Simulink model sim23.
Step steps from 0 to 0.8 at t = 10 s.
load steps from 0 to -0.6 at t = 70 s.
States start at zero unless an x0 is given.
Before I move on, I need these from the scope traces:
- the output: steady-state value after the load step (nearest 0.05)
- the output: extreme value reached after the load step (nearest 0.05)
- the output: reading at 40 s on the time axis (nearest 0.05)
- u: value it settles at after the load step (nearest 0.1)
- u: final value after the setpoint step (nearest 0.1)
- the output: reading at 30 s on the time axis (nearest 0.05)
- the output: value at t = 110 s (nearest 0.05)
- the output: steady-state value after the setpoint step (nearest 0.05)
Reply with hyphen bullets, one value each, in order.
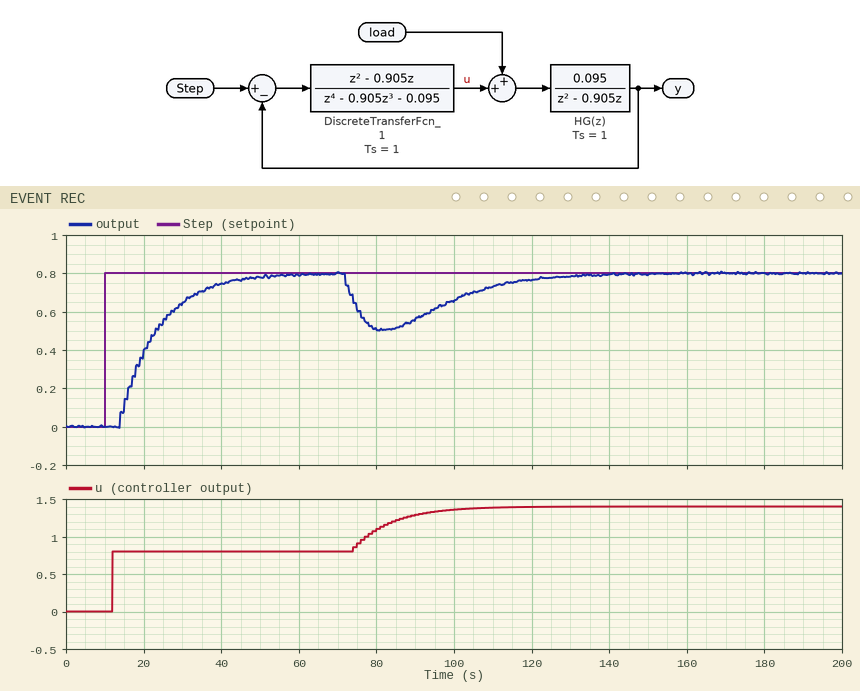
- 0.80
- 0.50
- 0.75
- 1.4
- 0.8
- 0.65
- 0.75
- 0.80
